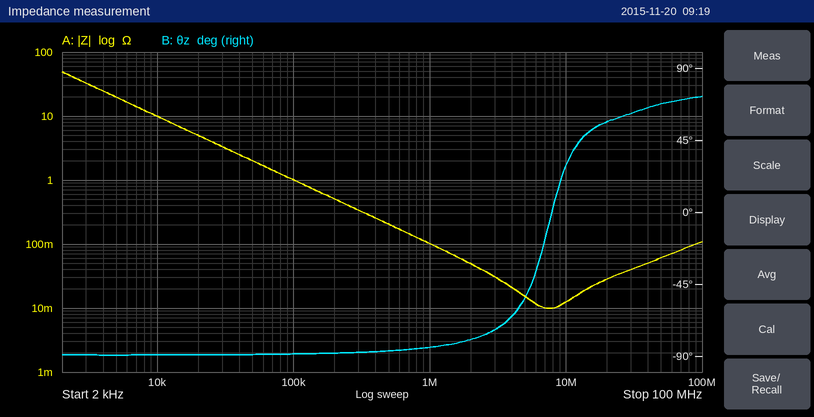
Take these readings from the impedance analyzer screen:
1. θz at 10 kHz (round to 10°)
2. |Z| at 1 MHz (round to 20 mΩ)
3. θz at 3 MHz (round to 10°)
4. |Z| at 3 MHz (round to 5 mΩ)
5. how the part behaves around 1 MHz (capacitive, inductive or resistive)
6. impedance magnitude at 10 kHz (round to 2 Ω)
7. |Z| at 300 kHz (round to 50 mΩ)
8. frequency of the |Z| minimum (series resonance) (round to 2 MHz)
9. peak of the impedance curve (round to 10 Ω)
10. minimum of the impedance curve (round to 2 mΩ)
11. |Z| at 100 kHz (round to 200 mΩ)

-90°
100 mΩ
-70°
30 mΩ
capacitive
10 Ω
350 mΩ
8 MHz
50 Ω
10 mΩ
1.0 Ω
